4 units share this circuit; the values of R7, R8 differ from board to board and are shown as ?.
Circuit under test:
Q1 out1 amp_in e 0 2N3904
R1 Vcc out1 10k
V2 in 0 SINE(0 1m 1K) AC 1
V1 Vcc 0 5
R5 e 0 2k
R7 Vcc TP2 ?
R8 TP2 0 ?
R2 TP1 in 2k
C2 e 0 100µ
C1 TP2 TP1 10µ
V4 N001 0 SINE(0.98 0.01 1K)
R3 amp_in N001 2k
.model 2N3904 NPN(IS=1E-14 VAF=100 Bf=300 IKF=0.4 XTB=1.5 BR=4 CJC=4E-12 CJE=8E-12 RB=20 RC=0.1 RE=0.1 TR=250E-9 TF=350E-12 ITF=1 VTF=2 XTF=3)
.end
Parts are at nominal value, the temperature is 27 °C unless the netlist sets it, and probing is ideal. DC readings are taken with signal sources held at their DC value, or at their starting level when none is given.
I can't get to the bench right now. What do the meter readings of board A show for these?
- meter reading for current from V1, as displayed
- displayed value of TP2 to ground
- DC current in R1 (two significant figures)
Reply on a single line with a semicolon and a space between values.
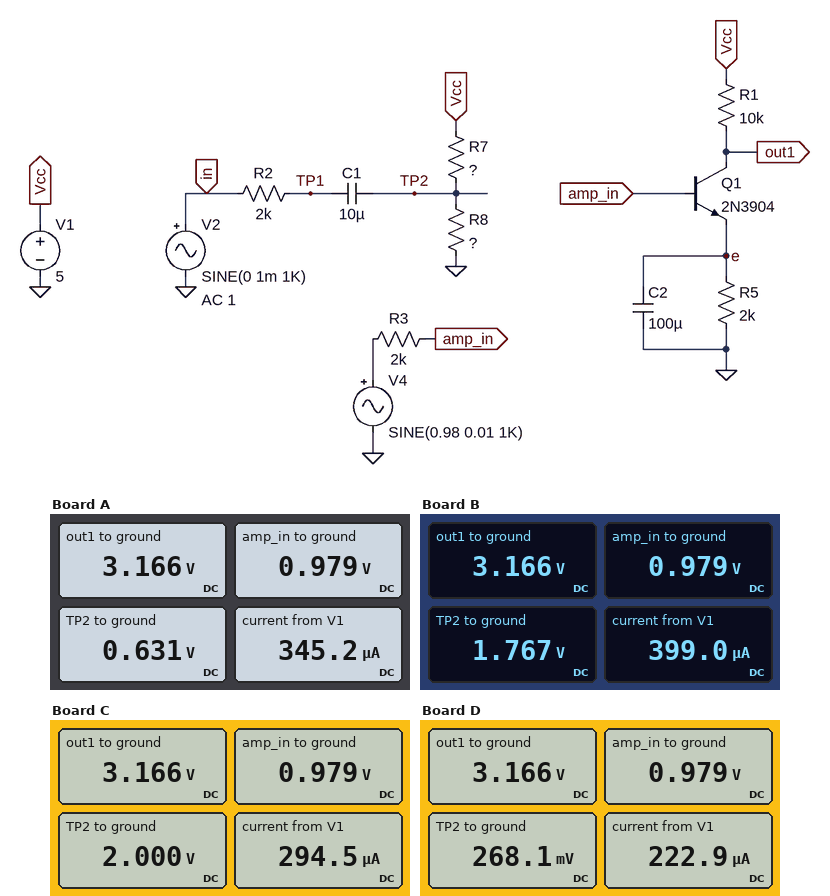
345.2 µA; 0.631 V; 180 µA
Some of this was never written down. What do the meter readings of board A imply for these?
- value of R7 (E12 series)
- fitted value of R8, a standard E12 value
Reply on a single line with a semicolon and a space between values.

27 kΩ; 3.9 kΩ
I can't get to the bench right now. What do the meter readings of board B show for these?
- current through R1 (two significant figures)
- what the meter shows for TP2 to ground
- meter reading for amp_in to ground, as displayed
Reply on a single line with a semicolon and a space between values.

180 µA; 1.767 V; 0.979 V
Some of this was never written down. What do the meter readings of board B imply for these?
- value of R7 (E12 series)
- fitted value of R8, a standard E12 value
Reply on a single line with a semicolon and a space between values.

15 kΩ; 8.2 kΩ
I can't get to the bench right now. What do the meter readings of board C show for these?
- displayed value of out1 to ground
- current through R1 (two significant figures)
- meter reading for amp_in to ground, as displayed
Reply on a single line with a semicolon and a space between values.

3.166 V; 180 µA; 0.979 V
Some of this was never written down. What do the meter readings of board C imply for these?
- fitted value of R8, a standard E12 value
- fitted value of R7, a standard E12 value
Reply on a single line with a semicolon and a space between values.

18 kΩ; 27 kΩ
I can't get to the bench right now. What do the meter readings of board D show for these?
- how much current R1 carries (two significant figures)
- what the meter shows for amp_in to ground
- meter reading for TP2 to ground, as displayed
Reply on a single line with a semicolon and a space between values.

180 µA; 0.979 V; 268.1 mV
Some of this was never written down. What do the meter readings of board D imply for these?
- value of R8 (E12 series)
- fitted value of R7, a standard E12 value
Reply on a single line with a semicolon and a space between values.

6.8 kΩ; 120 kΩ
